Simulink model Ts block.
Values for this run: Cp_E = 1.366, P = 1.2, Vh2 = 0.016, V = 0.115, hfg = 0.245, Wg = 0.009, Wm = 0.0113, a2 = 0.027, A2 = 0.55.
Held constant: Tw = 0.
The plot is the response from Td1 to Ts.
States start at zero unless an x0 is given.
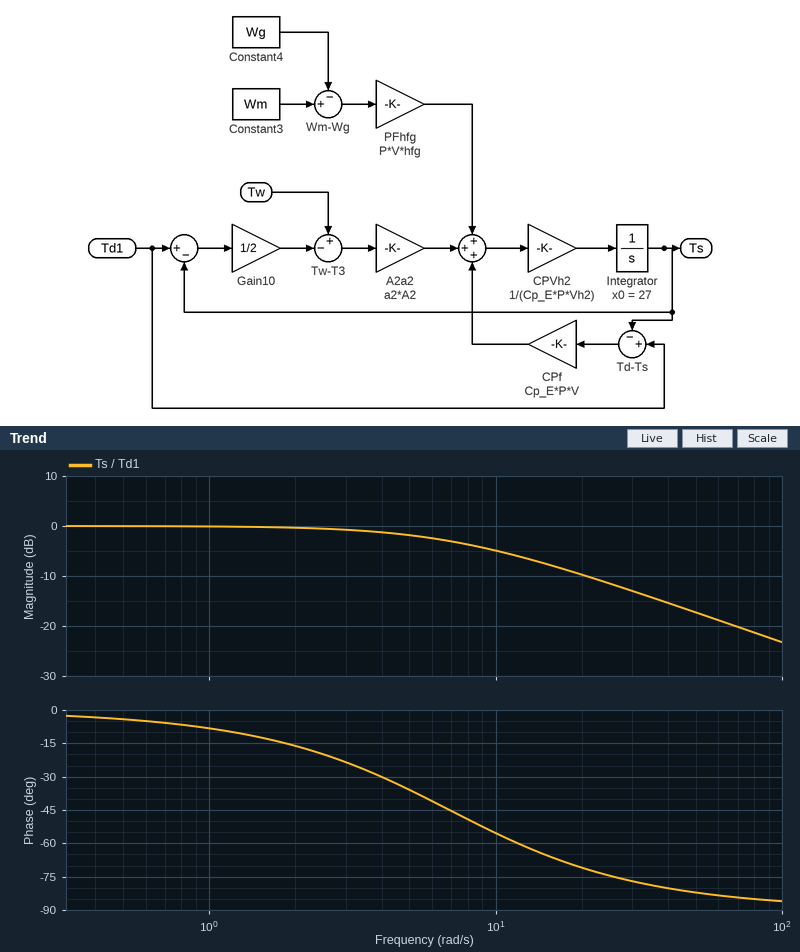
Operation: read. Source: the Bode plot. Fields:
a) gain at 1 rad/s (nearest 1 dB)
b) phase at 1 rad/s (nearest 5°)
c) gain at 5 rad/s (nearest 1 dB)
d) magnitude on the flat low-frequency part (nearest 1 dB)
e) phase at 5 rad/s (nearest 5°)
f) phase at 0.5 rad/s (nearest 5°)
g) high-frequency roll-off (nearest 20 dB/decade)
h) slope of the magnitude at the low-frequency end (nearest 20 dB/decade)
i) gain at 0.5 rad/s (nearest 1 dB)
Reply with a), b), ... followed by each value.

a) 0 dB
b) -10°
c) -2 dB
d) 0 dB
e) -35°
f) -5°
g) -20 dB/decade
h) 0 dB/decade
i) 0 dB
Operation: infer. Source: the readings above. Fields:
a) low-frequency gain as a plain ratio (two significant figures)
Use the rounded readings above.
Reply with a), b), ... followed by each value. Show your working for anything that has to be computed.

a) 10^(0 / 20) = 1.0
